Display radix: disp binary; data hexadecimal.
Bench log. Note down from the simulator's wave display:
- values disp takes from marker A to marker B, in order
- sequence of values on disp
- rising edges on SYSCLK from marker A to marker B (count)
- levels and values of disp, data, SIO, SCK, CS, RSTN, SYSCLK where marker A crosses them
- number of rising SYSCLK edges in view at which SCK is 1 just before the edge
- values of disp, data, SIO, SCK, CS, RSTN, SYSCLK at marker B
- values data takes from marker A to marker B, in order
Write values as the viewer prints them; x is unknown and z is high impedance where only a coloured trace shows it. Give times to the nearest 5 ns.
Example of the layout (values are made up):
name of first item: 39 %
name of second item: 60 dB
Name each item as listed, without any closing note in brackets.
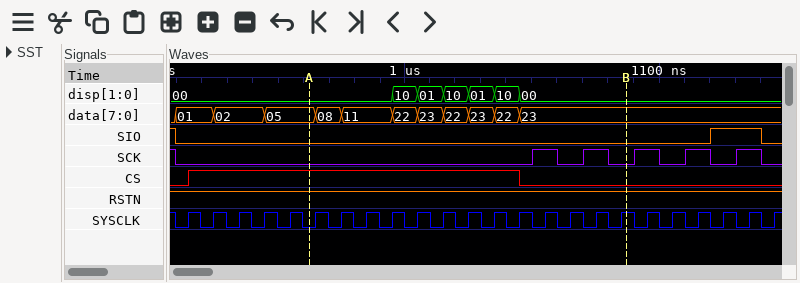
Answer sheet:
values disp takes from marker A to marker B, in order: 00, 10, 01, 10, 01, 10, 00
sequence of values on disp: 00, 10, 01, 10, 01, 10, 00
rising edges on SYSCLK from marker A to marker B: 13
levels and values of disp, data, SIO, SCK, CS, RSTN, SYSCLK where marker A crosses them: disp=00, data=05, SIO=0, SCK=0, CS=1, RSTN=1, SYSCLK=0
number of rising SYSCLK edges in view at which SCK is 1 just before the edge: 5
values of disp, data, SIO, SCK, CS, RSTN, SYSCLK at marker B: disp=00, data=23, SIO=0, SCK=0, CS=0, RSTN=1, SYSCLK=1
values data takes from marker A to marker B, in order: 05, 08, 11, 22, 23, 22, 23, 22, 23
